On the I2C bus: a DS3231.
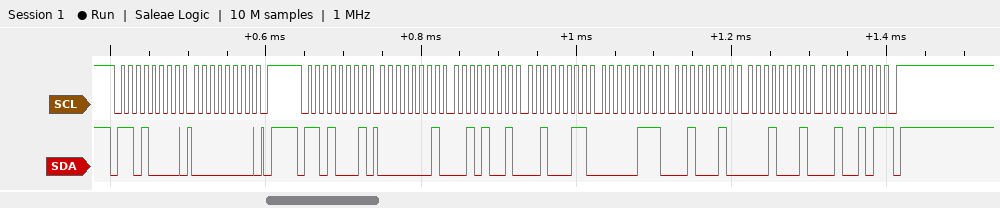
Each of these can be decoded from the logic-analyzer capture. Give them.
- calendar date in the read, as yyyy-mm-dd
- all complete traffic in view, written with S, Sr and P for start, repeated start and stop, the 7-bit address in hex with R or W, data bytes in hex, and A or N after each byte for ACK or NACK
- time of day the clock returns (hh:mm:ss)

2025-11-22
S 68W A 00 A P S 68R A 01 A 29 A 23 A 07 A 22 A 11 A 25 N P
23:29:01
